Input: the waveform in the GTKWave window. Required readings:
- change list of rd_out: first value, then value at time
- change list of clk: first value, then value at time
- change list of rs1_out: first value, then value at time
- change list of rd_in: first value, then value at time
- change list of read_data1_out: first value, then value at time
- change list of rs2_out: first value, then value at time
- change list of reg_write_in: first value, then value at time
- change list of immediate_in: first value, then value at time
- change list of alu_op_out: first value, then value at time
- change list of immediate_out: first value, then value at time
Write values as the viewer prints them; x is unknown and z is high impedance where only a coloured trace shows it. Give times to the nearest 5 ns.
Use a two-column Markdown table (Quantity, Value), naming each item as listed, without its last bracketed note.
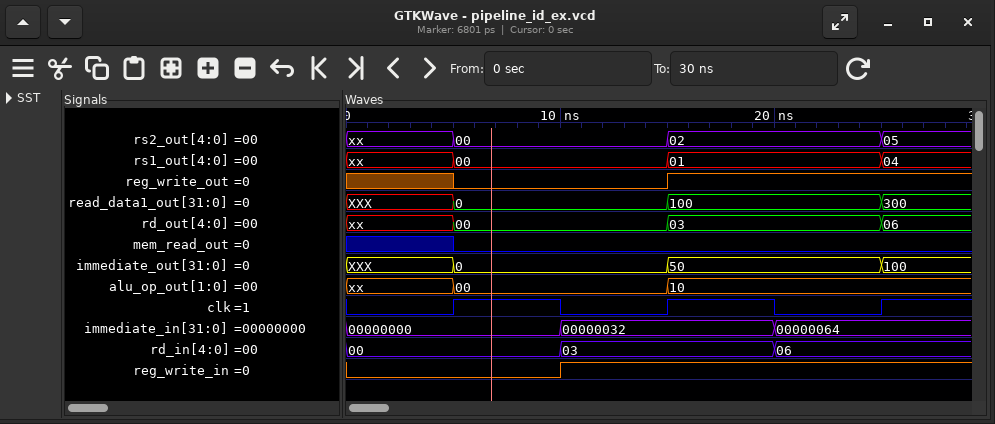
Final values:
| Quantity | Value |
|---|---|
| change list of rd_out: first value, then value at time | xx, 00 at 5 ns, 03 at 15 ns, 06 at 25 ns |
| change list of clk: first value, then value at time | 0, 1 at 5 ns, 0 at 10 ns, 1 at 15 ns, 0 at 20 ns, 1 at 25 ns |
| change list of rs1_out: first value, then value at time | xx, 00 at 5 ns, 01 at 15 ns, 04 at 25 ns |
| change list of rd_in: first value, then value at time | 00, 03 at 10 ns, 06 at 20 ns |
| change list of read_data1_out: first value, then value at time | XXX, 0 at 5 ns, 100 at 15 ns, 300 at 25 ns |
| change list of rs2_out: first value, then value at time | xx, 00 at 5 ns, 02 at 15 ns, 05 at 25 ns |
| change list of reg_write_in: first value, then value at time | 0, 1 at 10 ns |
| change list of immediate_in: first value, then value at time | 00000000, 00000032 at 10 ns, 00000064 at 20 ns |
| change list of alu_op_out: first value, then value at time | xx, 00 at 5 ns, 10 at 15 ns |
| change list of immediate_out: first value, then value at time | XXX, 0 at 5 ns, 50 at 15 ns, 100 at 25 ns |
